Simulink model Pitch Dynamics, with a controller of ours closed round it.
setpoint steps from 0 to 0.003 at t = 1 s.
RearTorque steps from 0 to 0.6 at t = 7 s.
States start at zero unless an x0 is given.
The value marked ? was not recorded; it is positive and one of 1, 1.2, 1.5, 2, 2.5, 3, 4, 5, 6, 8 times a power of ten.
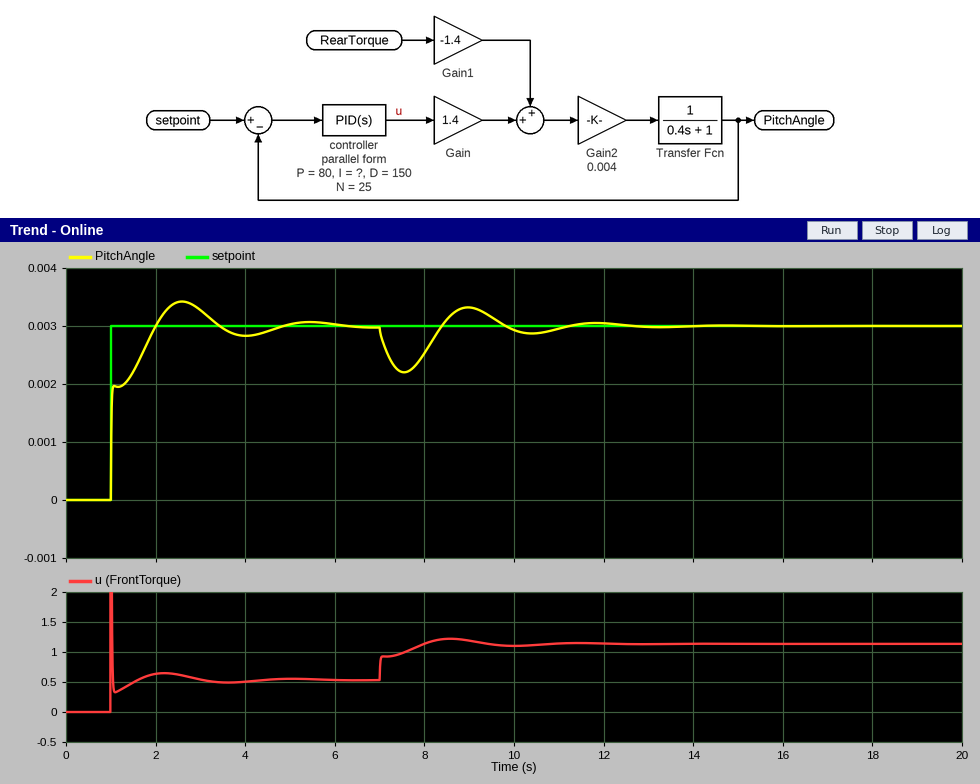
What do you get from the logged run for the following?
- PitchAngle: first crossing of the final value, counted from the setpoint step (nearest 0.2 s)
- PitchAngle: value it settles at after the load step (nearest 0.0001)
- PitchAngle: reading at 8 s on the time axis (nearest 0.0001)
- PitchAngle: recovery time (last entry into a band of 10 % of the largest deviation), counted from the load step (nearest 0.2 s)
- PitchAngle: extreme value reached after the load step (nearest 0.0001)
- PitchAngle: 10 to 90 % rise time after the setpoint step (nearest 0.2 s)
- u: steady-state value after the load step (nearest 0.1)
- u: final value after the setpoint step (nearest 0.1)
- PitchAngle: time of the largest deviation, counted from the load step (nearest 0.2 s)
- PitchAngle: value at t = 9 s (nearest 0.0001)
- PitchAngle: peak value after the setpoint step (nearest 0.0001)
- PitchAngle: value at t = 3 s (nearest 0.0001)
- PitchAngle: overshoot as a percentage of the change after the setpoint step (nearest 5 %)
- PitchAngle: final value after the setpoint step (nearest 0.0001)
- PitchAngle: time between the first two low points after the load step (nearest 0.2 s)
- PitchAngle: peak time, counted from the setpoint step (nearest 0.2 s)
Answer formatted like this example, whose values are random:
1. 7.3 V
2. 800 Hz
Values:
1. 1.0 s
2. 0.0030
3. 0.0025
4. 3.8 s
5. 0.0022
6. 0.8 s
7. 1.1
8. 0.5
9. 0.6 s
10. 0.0033
11. 0.0034
12. 0.0033
13. 15 %
14. 0.0030
15. 2.8 s
16. 1.6 s
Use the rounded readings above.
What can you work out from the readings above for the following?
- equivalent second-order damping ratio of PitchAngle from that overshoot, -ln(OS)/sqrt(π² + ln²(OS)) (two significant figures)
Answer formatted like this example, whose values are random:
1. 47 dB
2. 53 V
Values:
1. 0.52
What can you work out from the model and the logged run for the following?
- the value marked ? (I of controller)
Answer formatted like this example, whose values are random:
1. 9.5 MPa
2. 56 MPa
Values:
1. 1200
